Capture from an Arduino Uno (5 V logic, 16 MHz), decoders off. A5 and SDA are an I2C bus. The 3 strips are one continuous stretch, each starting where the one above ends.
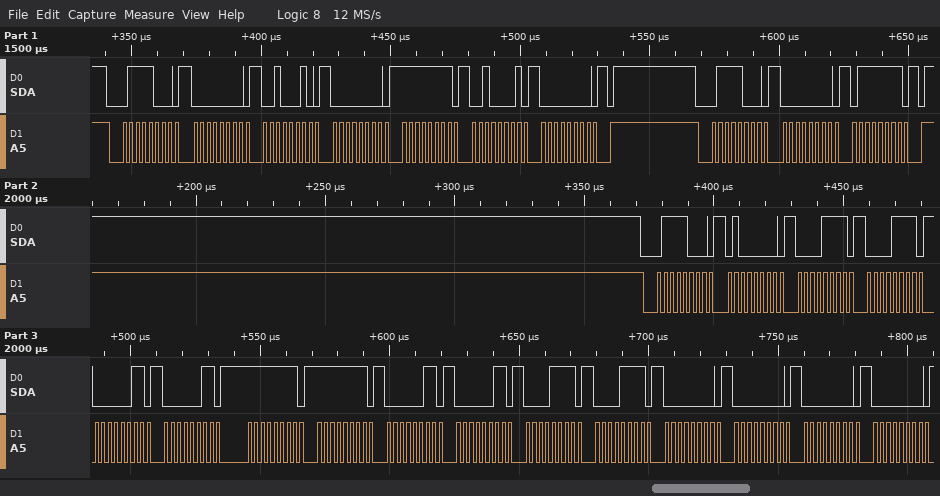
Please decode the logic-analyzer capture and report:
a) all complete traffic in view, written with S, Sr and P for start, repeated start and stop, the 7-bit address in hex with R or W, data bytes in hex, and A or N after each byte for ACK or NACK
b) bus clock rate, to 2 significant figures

S 3CW A 00 A 22 A 00 A FF A 21 A 00 A P S 3CW A 00 A 7F A P S 3CW A 40 A 0F A 0F A 03 A 03 A FF A FF A 03 A 03 A 0F A 0F A 00 A 00 A 00 A 00 A
400 kHz
